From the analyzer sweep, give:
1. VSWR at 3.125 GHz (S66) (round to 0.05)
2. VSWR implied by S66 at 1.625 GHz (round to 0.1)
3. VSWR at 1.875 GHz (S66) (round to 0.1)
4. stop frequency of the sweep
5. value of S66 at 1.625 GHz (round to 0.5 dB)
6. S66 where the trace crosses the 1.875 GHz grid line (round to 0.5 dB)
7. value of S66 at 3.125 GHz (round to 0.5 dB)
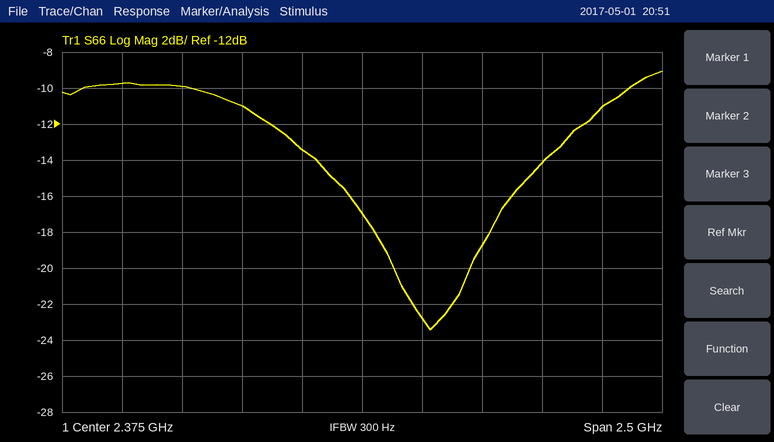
1.50
1.9
1.8
3.625 GHz
-10.0 dB
-11.0 dB
-14.0 dB
